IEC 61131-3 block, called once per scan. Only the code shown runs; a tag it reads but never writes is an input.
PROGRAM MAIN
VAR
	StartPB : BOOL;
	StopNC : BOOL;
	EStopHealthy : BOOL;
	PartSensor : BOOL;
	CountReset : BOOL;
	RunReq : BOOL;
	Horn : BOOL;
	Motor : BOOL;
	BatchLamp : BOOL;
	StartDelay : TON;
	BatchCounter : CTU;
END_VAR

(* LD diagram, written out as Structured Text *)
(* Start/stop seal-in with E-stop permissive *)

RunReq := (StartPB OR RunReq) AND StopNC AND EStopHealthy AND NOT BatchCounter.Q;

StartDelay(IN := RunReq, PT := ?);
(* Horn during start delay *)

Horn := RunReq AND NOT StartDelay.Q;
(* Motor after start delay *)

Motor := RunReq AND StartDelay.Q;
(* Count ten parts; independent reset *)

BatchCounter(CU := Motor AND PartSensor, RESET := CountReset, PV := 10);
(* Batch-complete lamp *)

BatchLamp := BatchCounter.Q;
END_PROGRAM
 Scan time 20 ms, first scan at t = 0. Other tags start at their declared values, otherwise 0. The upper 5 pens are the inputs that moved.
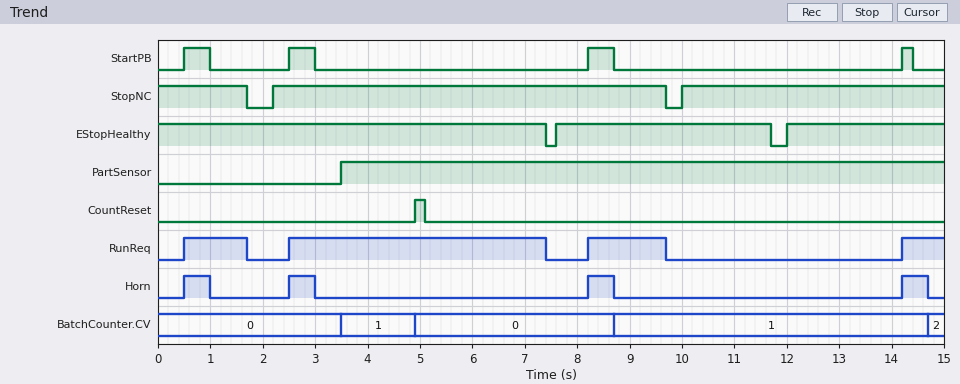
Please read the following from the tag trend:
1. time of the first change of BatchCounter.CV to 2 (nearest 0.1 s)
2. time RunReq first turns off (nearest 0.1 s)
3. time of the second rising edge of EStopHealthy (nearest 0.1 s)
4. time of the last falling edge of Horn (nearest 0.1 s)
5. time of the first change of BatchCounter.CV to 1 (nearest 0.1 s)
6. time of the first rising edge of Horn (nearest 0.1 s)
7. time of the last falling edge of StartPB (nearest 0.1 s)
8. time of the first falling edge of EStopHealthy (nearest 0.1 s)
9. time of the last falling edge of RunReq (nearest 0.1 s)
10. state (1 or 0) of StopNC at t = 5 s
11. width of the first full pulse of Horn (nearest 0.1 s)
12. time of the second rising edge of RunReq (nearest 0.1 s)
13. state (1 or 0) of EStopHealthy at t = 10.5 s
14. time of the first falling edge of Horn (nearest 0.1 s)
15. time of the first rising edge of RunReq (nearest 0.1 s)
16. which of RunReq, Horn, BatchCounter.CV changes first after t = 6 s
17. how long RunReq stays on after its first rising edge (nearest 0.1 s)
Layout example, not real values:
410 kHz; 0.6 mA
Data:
14.7 s; 1.7 s; 12.0 s; 14.7 s; 3.5 s; 0.5 s; 14.4 s; 7.4 s; 9.7 s; 1; 0.5 s; 2.5 s; 1; 1.0 s; 0.5 s; RunReq; 1.2 s
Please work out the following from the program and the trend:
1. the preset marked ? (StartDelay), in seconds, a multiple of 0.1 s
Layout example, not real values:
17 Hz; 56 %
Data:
0.5 s
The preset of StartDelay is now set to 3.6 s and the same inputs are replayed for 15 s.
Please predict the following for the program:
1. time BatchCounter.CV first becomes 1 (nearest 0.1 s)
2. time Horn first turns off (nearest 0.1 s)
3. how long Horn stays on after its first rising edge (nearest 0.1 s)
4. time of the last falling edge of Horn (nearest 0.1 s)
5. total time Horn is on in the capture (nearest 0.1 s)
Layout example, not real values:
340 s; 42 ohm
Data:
6.1 s; 1.7 s; 1.2 s; 9.7 s; 7.1 s
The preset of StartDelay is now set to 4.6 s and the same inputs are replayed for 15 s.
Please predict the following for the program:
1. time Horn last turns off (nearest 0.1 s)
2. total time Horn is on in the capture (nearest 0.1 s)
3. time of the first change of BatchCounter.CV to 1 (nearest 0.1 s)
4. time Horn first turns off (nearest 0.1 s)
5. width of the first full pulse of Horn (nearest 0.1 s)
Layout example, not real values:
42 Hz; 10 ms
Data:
9.7 s; 8.1 s; 7.1 s; 1.7 s; 1.2 s
